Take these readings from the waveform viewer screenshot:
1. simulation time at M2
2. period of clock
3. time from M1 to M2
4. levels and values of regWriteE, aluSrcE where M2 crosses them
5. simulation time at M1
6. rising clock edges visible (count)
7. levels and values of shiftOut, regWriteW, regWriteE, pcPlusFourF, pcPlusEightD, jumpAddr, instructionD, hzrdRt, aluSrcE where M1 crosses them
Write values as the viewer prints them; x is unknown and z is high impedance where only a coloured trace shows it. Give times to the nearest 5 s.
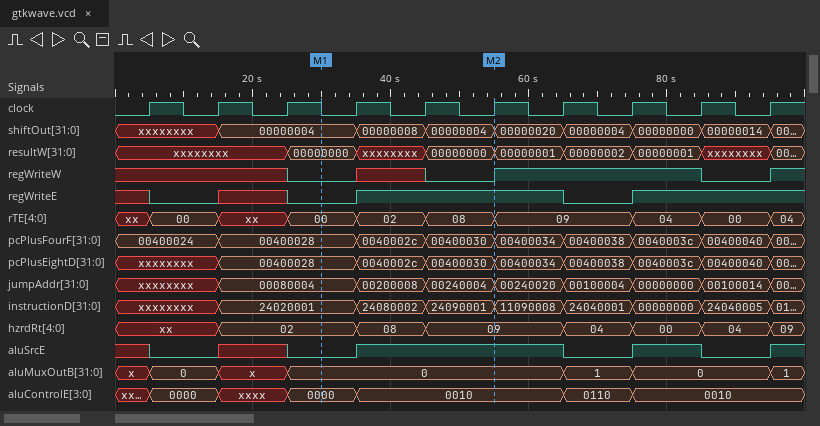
55 s
10 s
25 s
regWriteE=1, aluSrcE=1
30 s
10
shiftOut=00000004, regWriteW=0, regWriteE=0, pcPlusFourF=00400028, pcPlusEightD=00400028, jumpAddr=00080004, instructionD=24020001, hzrdRt=02, aluSrcE=0
